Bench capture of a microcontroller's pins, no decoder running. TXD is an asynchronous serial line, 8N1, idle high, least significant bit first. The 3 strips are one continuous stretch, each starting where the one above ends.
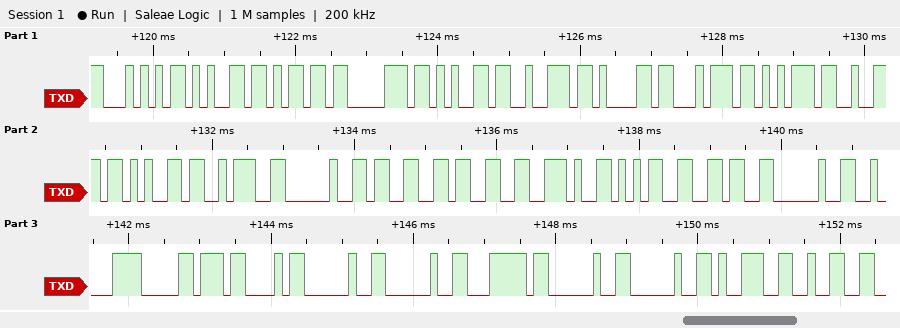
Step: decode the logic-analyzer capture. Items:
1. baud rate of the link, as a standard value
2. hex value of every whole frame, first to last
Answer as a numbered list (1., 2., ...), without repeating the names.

1. 9600 baud
2. 54 65 6D 70 65 72 61 74 75 72 65 3A 20 33 33 2E 35 36 20 C2 B0 43 20 20 7C 20 20 39 32
